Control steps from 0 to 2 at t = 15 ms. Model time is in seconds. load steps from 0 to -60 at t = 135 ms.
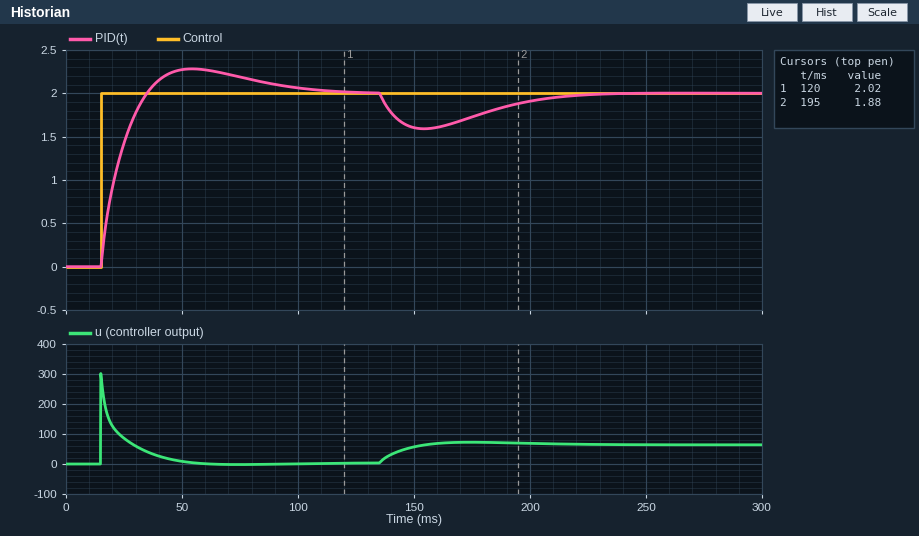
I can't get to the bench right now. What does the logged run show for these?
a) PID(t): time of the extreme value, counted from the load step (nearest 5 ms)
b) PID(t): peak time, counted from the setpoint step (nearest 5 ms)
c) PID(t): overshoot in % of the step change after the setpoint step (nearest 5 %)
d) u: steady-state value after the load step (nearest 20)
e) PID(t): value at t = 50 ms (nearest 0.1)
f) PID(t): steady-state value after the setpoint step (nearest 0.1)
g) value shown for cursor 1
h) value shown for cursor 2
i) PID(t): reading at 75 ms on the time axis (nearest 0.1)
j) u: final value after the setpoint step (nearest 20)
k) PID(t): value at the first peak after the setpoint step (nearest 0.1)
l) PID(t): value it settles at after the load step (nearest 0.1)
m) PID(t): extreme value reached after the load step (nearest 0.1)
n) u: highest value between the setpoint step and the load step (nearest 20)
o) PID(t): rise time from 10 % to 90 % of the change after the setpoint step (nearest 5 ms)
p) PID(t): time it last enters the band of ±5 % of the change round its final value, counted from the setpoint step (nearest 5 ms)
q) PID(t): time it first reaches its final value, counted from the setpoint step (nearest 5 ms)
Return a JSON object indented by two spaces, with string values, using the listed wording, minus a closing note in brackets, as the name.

{
  "PID(t): time of the extreme value, counted from the load step": "20 ms",
  "PID(t): peak time, counted from the setpoint step": "40 ms",
  "PID(t): overshoot in % of the step change after the setpoint step": "15 %",
  "u: steady-state value after the load step": "60",
  "PID(t): value at t = 50 ms": "2.3",
  "PID(t): steady-state value after the setpoint step": "2.0",
  "value shown for cursor 1": "2.02",
  "value shown for cursor 2": "1.88",
  "PID(t): reading at 75 ms on the time axis": "2.2",
  "u: final value after the setpoint step": "0",
  "PID(t): value at the first peak after the setpoint step": "2.3",
  "PID(t): value it settles at after the load step": "2.0",
  "PID(t): extreme value reached after the load step": "1.6",
  "u: highest value between the setpoint step and the load step": "300",
  "PID(t): rise time from 10 % to 90 % of the change after the setpoint step": "15 ms",
  "PID(t): time it last enters the band of ±5 % of the change round its final value, counted from the setpoint step": "75 ms",
  "PID(t): time it first reaches its final value, counted from the setpoint step": "20 ms"
}
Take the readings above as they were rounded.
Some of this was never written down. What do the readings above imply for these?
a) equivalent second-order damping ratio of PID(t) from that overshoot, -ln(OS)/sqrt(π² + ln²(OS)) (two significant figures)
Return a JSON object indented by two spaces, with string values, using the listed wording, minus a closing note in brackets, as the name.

{
  "equivalent second-order damping ratio of PID(t) from that overshoot, -ln(OS)/sqrt(π² + ln²(OS))": "0.52"
}
